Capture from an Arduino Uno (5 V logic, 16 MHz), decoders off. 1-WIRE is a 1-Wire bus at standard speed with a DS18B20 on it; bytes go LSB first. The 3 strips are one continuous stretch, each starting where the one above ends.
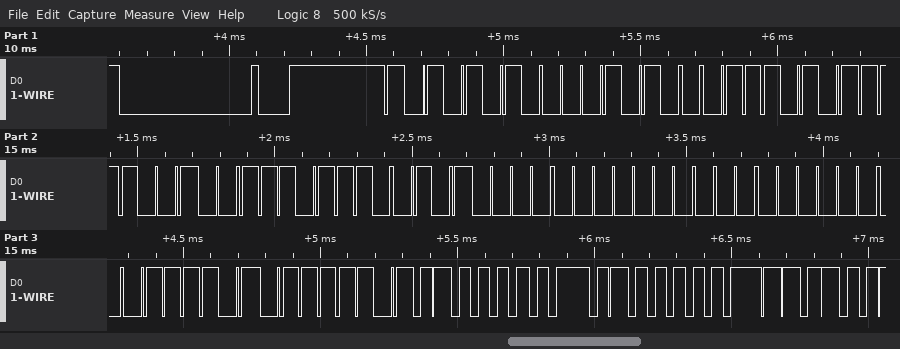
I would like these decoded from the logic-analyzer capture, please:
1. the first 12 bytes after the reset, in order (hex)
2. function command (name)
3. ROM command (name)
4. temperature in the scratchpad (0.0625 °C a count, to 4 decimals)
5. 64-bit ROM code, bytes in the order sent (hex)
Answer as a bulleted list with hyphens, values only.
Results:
- 55 28 AE 27 77 0A 00 00 BC BE 02 02
- Read Scratchpad
- Match ROM
- 32.1250 °C
- 28 AE 27 77 0A 00 00 BC
